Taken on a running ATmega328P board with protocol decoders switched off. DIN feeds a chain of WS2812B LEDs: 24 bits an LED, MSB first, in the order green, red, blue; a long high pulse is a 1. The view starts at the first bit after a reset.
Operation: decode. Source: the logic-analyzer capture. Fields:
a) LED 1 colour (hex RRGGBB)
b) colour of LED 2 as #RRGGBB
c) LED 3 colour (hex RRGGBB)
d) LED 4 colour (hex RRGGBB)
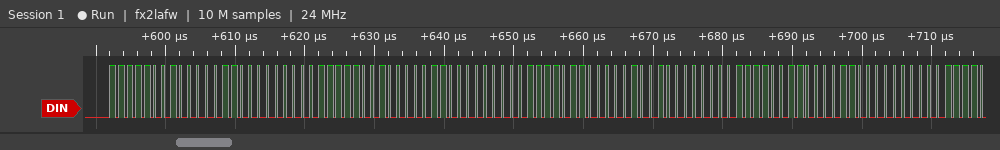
#06F900
#06F900
#09F600
#0CF300
